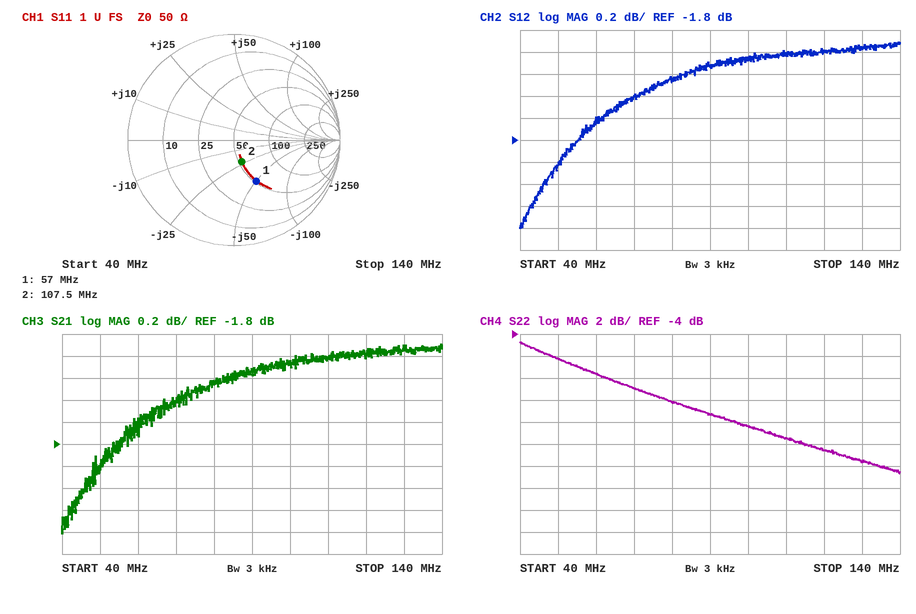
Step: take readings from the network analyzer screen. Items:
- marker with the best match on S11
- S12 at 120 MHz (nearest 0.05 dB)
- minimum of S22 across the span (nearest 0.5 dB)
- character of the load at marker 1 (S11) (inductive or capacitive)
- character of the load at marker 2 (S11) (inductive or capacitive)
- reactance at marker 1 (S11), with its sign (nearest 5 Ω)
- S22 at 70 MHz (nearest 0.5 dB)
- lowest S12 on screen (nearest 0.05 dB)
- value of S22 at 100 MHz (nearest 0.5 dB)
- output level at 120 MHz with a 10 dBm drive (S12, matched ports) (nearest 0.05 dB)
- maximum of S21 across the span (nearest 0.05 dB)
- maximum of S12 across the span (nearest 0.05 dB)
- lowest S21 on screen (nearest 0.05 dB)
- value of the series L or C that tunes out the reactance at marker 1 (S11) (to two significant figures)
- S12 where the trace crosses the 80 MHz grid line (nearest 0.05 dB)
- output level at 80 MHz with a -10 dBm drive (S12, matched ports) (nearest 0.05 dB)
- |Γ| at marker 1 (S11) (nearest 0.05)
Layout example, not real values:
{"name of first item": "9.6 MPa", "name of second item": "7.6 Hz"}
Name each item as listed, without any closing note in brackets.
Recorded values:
{"marker with the best match on S11": "marker 2", "S12 at 120 MHz": "-1.00 dB", "minimum of S22 across the span": "-16.5 dB", "character of the load at marker 1 (S11)": "capacitive", "character of the load at marker 2 (S11)": "capacitive", "reactance at marker 1 (S11), with its sign": "-50 Ω", "S22 at 70 MHz": "-9.0 dB", "lowest S12 on screen": "-2.60 dB", "value of S22 at 100 MHz": "-12.5 dB", "output level at 120 MHz with a 10 dBm drive (S12, matched ports)": "9.00 dBm", "maximum of S21 across the span": "-0.90 dB", "maximum of S12 across the span": "-0.90 dB", "lowest S21 on screen": "-2.60 dB", "value of the series L or C that tunes out the reactance at marker 1 (S11)": "140 nH", "S12 where the trace crosses the 80 MHz grid line": "-1.25 dB", "output level at 80 MHz with a -10 dBm drive (S12, matched ports)": "-11.25 dBm", "|Γ| at marker 1 (S11)": "0.45"}
